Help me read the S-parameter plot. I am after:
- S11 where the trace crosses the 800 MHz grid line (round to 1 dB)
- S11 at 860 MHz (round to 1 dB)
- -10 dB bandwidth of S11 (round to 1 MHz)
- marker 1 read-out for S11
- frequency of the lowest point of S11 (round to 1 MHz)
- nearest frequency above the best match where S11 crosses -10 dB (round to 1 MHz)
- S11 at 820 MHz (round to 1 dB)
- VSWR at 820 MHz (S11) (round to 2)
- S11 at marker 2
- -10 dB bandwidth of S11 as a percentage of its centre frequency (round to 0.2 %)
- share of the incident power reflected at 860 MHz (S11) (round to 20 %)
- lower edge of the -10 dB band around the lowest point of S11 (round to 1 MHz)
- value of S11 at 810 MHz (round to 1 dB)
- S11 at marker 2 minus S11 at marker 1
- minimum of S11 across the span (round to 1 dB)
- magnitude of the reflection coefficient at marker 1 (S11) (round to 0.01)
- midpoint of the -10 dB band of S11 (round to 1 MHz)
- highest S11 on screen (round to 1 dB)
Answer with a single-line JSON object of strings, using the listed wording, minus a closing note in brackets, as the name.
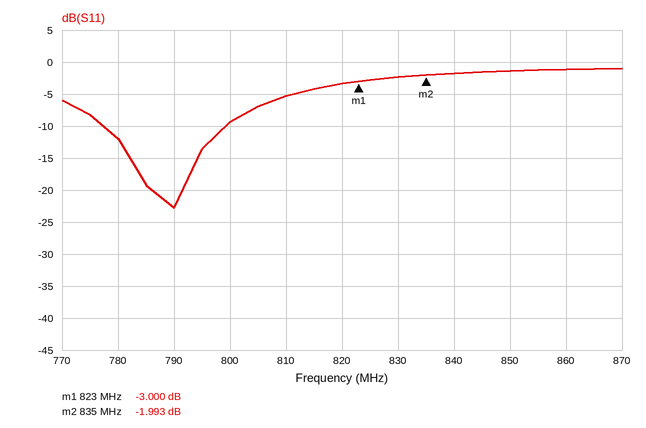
{"S11 where the trace crosses the 800 MHz grid line": "-9 dB", "S11 at 860 MHz": "-1 dB", "-10 dB bandwidth of S11": "22 MHz", "marker 1 read-out for S11": "-3.000 dB", "frequency of the lowest point of S11": "790 MHz", "nearest frequency above the best match where S11 crosses -10 dB": "799 MHz", "S11 at 820 MHz": "-3 dB", "VSWR at 820 MHz (S11)": "6", "S11 at marker 2": "-1.993 dB", "-10 dB bandwidth of S11 as a percentage of its centre frequency": "2.8 %", "share of the incident power reflected at 860 MHz (S11)": "80 %", "lower edge of the -10 dB band around the lowest point of S11": "777 MHz", "value of S11 at 810 MHz": "-5 dB", "S11 at marker 2 minus S11 at marker 1": "1.007 dB", "minimum of S11 across the span": "-23 dB", "magnitude of the reflection coefficient at marker 1 (S11)": "0.71", "midpoint of the -10 dB band of S11": "788 MHz", "highest S11 on screen": "-1 dB"}
